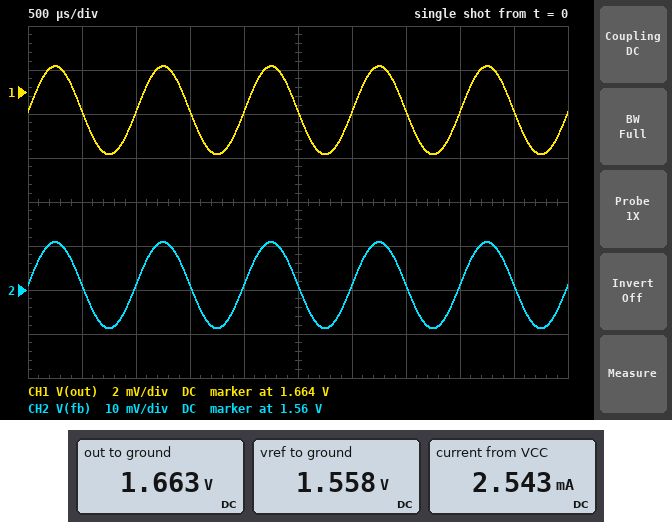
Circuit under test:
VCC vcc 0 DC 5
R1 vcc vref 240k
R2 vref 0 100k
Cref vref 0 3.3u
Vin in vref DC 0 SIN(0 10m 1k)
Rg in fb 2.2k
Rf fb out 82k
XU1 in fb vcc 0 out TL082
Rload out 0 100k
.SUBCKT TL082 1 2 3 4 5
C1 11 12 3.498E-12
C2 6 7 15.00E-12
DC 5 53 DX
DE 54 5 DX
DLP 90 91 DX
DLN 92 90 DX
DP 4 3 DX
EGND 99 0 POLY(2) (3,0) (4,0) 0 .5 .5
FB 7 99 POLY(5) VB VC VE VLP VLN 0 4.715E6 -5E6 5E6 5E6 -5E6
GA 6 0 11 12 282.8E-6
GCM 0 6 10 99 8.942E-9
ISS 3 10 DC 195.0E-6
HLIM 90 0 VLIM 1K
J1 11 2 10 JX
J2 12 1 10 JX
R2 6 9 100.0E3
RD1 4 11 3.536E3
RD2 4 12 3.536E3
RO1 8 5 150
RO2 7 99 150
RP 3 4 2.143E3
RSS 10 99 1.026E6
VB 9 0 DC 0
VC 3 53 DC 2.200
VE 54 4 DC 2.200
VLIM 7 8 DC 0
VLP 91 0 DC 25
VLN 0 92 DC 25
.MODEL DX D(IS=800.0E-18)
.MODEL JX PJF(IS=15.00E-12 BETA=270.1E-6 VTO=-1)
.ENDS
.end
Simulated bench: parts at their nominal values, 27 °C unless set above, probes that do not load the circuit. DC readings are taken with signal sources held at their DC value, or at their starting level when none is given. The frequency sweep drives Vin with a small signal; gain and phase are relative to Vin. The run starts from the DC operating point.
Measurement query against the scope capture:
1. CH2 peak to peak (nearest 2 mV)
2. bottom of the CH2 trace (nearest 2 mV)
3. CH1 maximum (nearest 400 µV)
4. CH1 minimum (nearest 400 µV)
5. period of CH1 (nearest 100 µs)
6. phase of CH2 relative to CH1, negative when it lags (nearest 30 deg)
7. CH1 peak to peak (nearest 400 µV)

20 mV
1.552 V
1.6652 V
1.6612 V
1.0 ms
0 deg
4.0 mV
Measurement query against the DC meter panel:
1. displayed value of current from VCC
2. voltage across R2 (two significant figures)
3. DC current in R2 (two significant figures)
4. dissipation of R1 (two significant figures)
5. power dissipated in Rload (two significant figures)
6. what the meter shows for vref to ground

2.543 mA
1.6 V
16 µA
49 µW
28 µW
1.558 V
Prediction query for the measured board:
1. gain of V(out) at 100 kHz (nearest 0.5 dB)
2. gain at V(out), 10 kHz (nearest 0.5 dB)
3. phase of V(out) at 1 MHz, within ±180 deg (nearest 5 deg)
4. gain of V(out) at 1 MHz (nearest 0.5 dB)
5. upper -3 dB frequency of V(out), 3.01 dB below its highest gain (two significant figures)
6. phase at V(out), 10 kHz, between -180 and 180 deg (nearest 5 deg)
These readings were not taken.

-17.0 dB
-14.0 dB
-90 deg
-34.0 dB
100 kHz
-5 deg
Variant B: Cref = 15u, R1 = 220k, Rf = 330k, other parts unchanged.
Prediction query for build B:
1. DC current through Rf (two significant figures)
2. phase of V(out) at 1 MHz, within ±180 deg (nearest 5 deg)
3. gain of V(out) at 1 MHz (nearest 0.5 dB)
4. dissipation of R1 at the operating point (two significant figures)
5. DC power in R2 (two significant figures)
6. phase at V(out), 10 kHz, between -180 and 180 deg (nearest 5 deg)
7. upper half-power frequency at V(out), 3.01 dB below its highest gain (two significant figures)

340 nA
-95 deg
-38.5 dB
53 µW
25 µW
-10 deg
62 kHz
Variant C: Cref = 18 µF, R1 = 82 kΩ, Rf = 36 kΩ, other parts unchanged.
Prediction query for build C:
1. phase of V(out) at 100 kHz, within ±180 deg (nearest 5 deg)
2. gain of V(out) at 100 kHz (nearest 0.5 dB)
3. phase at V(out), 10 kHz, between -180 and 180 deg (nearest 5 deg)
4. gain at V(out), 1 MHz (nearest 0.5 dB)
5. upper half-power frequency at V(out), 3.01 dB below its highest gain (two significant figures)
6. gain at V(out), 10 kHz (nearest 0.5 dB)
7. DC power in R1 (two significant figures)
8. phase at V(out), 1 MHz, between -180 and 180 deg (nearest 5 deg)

-25 deg
-1.0 dB
-5 deg
-14.0 dB
200 kHz
0 dB
62 µW
-85 deg
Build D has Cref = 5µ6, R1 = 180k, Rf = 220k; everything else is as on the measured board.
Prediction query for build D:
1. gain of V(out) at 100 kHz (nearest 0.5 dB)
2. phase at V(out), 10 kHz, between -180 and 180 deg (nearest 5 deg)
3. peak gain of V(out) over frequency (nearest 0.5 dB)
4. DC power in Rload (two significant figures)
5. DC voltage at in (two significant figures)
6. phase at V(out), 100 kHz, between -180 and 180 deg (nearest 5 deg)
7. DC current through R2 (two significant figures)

-10.0 dB
-15 deg
-0.5 dB
32 µW
1.8 V
-70 deg
18 µA
